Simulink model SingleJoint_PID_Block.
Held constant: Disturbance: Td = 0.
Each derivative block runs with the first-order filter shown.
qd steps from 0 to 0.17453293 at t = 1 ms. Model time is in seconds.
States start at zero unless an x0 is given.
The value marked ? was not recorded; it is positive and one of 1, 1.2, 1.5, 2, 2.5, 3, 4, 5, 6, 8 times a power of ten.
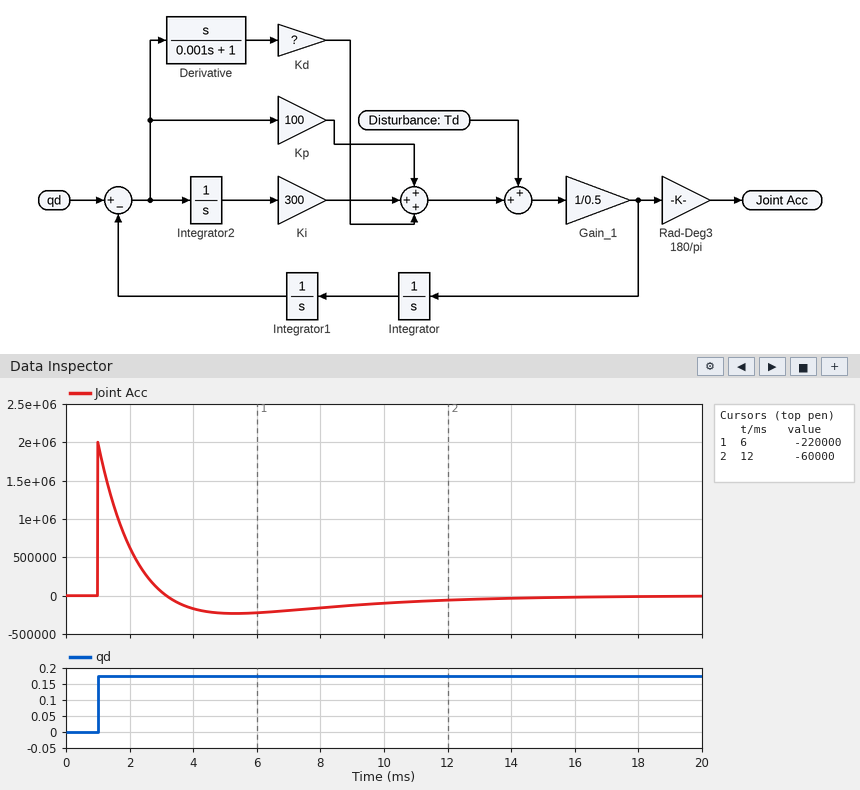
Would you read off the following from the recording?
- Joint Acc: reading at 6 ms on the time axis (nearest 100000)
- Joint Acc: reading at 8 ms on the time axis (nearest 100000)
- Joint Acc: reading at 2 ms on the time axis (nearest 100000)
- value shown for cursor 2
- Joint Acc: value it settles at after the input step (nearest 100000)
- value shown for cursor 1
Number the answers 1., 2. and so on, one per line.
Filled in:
1. -200000
2. -200000
3. 600000
4. -60000
5. 0
6. -220000
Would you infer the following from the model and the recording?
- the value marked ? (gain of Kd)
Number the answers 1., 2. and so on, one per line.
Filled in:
1. 100
